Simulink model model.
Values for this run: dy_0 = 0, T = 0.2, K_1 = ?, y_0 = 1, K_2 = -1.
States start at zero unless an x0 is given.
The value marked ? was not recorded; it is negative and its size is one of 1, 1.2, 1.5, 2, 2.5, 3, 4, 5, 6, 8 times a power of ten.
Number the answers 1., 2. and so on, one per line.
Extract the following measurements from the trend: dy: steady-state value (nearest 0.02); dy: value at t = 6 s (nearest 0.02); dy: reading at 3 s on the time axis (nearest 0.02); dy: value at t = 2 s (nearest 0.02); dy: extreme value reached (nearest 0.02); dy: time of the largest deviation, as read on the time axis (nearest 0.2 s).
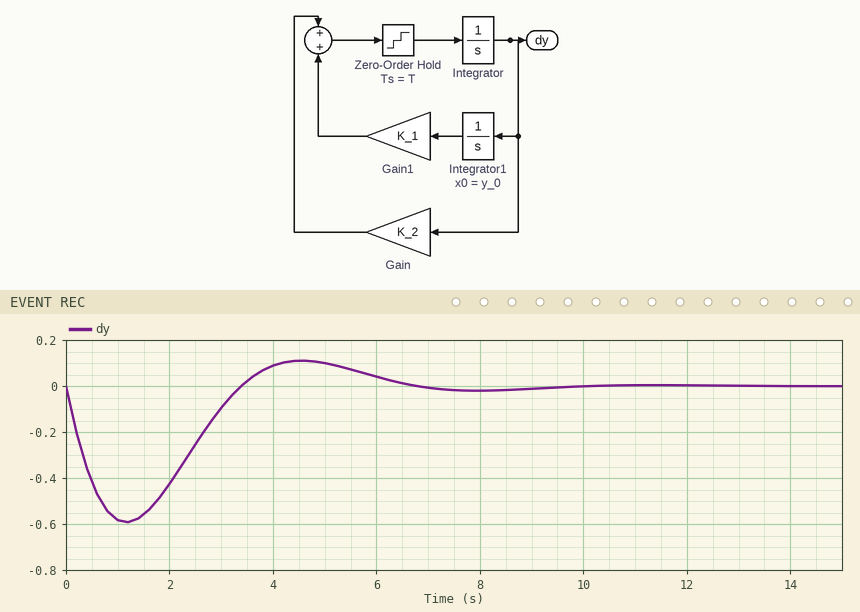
1. 0.00
2. 0.04
3. -0.10
4. -0.42
5. -0.60
6. 1.2 s
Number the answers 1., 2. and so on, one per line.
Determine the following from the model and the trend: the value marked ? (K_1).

1. -1
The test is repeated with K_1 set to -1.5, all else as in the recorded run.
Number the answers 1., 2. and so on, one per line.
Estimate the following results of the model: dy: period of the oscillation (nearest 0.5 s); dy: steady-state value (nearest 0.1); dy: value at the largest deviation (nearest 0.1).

1. 5.0 s
2. 0.0
3. -0.8
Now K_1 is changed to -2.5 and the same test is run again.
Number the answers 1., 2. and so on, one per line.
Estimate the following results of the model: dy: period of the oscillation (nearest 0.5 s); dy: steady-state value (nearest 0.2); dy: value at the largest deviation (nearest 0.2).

1. 4.0 s
2. 0.0
3. -1.2
